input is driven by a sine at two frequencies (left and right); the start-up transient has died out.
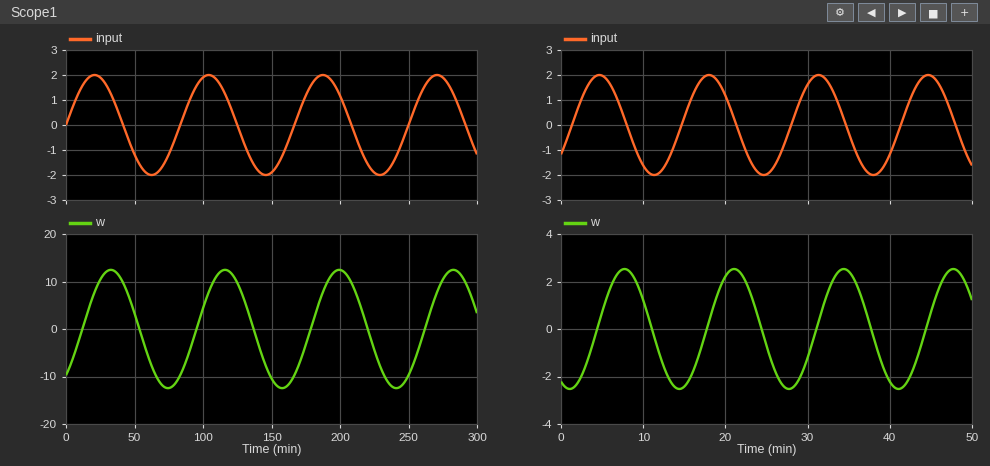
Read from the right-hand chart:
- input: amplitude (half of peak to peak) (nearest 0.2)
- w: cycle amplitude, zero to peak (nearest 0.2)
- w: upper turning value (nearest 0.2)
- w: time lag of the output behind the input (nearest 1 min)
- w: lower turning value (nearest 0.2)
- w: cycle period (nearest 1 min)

2.0
2.6
2.6
3 min
-2.6
13 min
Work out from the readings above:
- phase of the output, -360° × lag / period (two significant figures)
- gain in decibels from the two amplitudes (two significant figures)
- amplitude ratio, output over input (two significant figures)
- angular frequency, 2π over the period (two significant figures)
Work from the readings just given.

-83°
2.3 dB
1.3
0.48 rad/min
